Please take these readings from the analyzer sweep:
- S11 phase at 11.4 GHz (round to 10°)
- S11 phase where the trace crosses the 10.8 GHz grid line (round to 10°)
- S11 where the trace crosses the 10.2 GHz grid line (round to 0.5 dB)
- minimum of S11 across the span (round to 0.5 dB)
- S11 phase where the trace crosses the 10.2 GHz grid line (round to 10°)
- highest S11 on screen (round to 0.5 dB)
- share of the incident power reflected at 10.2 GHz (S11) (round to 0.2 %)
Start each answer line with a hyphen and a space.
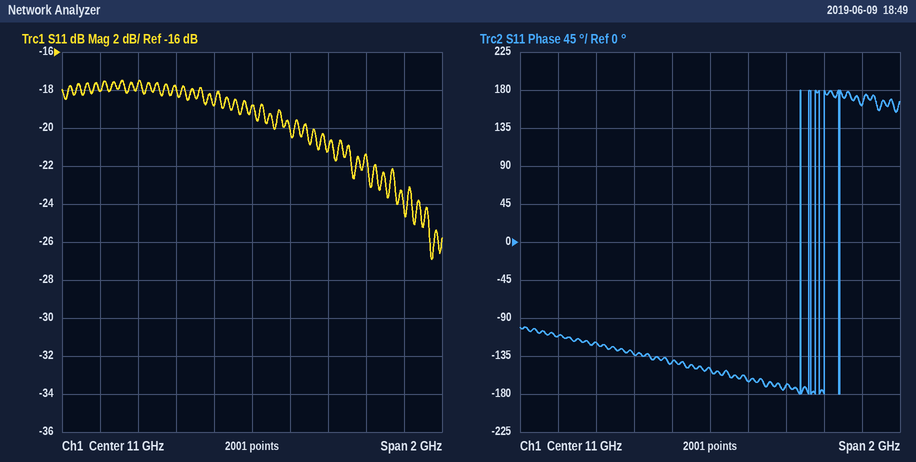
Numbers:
- -170°
- -140°
- -18.0 dB
- -27.0 dB
- -110°
- -17.5 dB
- 1.6 %
